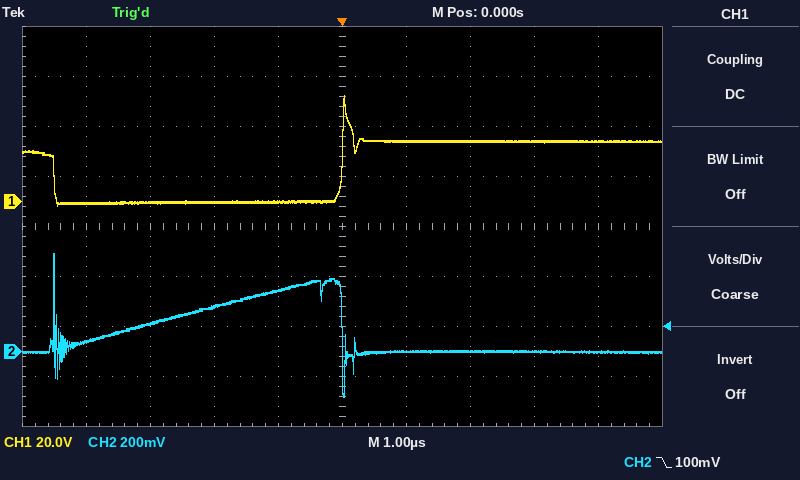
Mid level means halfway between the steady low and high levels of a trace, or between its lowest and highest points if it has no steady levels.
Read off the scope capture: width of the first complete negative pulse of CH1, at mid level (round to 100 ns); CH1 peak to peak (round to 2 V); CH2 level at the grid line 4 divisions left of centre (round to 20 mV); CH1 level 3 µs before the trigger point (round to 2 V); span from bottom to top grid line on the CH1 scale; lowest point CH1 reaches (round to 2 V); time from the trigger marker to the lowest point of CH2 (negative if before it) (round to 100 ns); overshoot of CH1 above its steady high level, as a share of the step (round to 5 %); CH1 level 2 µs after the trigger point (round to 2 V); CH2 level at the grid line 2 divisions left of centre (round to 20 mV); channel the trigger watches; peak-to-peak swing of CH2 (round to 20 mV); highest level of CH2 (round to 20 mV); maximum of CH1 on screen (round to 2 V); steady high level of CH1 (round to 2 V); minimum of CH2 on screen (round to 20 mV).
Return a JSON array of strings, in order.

["4.5 µs", "44 V", "40 mV", "0 V", "160 V", "-2 V", "0.0 µs", "75 %", "24 V", "180 mV", "CH2", "580 mV", "400 mV", "42 V", "24 V", "-180 mV"]
